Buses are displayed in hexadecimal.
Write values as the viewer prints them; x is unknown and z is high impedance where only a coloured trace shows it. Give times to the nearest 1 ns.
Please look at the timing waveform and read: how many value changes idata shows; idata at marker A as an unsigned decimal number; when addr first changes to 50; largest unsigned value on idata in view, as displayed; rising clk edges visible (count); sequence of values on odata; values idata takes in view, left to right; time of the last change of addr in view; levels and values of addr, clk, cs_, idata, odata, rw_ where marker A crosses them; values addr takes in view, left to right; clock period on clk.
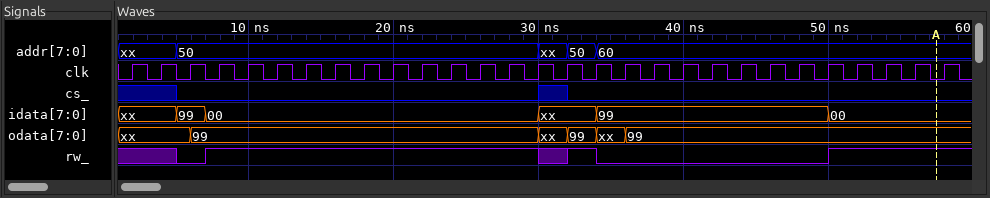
5
0
5 ns
99
29
xx, 99, xx, 99, xx, 99
xx, 99, 00, xx, 99, 00
34 ns
addr=60, clk=0, cs_=0, idata=00, odata=99, rw_=1
xx, 50, xx, 50, 60
2 ns
